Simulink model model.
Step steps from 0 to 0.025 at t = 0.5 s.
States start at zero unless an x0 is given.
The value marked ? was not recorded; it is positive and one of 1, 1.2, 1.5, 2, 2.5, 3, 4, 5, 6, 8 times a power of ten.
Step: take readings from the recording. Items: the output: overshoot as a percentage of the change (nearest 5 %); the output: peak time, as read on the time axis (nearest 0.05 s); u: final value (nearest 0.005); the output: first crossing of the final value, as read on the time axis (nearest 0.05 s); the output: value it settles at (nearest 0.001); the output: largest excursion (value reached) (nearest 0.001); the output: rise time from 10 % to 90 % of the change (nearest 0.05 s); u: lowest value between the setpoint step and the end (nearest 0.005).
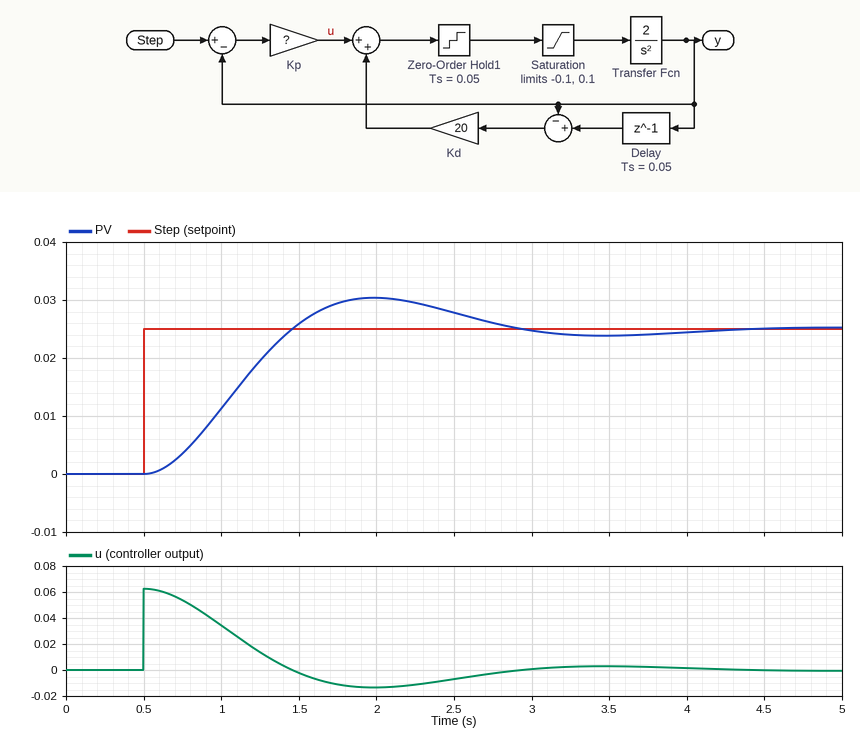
20 %
2.00 s
0.000
1.45 s
0.025
0.030
0.65 s
-0.015
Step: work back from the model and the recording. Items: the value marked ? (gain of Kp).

2.5
